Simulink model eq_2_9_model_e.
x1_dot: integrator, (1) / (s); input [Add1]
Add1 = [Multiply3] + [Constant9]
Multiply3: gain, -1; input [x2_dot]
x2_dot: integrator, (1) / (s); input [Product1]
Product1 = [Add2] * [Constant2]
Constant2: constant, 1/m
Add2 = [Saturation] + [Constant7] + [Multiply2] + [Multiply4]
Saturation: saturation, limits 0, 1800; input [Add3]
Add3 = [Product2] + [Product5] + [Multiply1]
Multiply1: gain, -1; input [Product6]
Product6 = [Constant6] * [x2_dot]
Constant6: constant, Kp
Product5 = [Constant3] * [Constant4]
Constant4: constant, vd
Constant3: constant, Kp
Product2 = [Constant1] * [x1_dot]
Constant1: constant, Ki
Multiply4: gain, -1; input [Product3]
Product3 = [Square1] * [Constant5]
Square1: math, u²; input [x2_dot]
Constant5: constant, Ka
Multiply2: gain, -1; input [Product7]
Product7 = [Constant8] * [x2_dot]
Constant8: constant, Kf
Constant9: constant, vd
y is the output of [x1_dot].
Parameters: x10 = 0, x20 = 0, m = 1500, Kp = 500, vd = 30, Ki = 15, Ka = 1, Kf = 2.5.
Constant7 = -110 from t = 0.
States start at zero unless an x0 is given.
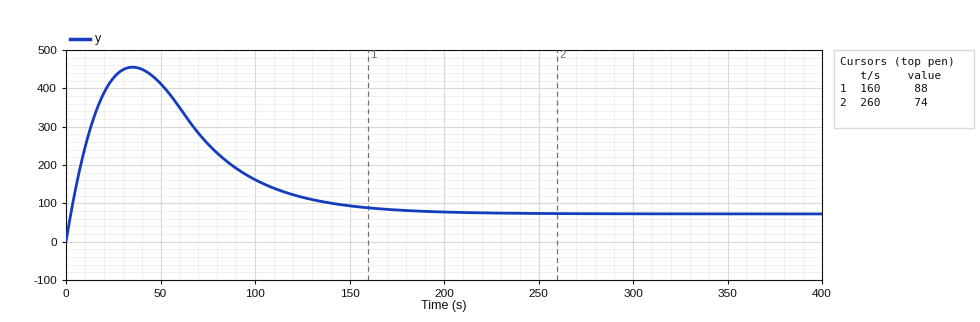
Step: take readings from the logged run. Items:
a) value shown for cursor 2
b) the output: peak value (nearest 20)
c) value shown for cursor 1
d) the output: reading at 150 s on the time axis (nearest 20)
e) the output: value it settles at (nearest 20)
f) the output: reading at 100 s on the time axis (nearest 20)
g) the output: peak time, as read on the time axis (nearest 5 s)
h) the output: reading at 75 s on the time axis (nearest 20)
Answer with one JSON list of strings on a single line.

["74", "460", "88", "100", "80", "160", "35 s", "260"]
